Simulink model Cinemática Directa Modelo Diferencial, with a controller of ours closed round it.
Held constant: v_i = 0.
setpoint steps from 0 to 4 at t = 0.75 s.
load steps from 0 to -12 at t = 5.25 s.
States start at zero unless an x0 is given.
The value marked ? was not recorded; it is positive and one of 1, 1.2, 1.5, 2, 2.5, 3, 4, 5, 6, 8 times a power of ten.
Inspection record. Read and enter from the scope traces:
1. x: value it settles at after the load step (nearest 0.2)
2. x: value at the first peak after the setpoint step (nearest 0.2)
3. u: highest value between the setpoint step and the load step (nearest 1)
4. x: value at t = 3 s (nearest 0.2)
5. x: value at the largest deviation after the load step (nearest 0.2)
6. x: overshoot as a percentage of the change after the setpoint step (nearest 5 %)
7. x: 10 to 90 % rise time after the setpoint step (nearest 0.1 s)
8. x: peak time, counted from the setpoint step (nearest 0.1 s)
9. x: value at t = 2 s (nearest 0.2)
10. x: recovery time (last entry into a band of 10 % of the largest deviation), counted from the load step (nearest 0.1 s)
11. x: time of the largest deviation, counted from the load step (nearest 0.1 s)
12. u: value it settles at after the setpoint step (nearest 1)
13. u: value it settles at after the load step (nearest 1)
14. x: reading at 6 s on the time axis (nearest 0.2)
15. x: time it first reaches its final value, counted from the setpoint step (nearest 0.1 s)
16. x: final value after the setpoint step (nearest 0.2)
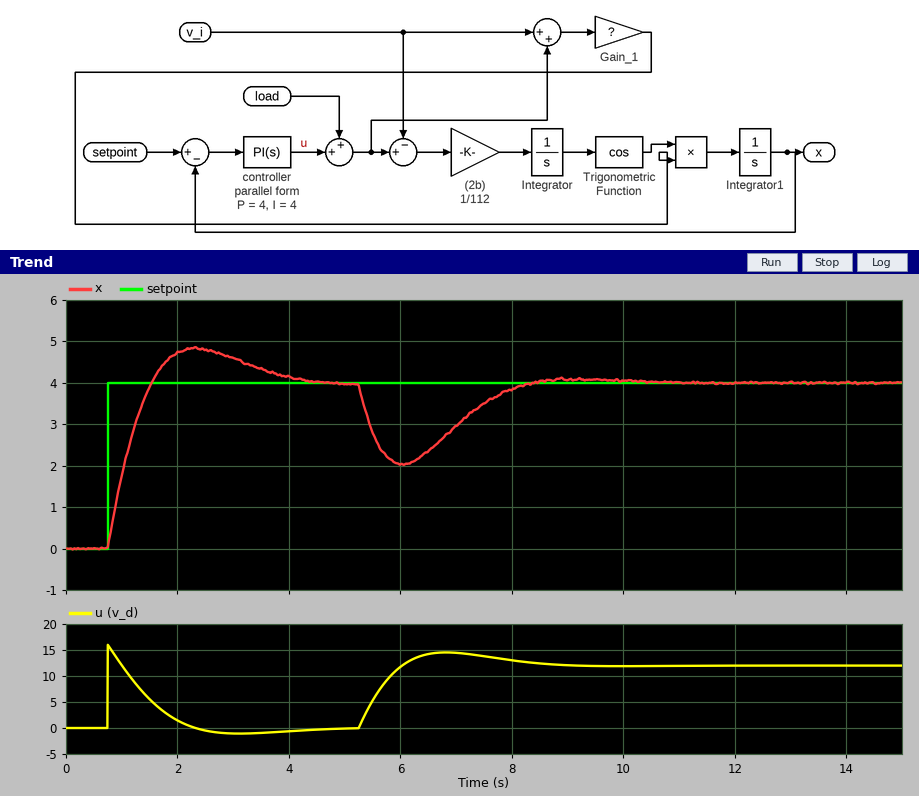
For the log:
4.0
4.8
16
4.6
2.0
20 %
0.6 s
1.6 s
4.8
2.7 s
0.8 s
0
12
2.0
0.8 s
4.0
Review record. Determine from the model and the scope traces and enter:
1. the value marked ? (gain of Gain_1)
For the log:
0.5
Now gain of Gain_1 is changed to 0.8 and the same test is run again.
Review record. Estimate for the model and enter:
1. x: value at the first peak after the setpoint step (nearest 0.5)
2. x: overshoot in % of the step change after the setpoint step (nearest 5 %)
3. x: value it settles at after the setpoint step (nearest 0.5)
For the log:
4.5
15 %
4.0
